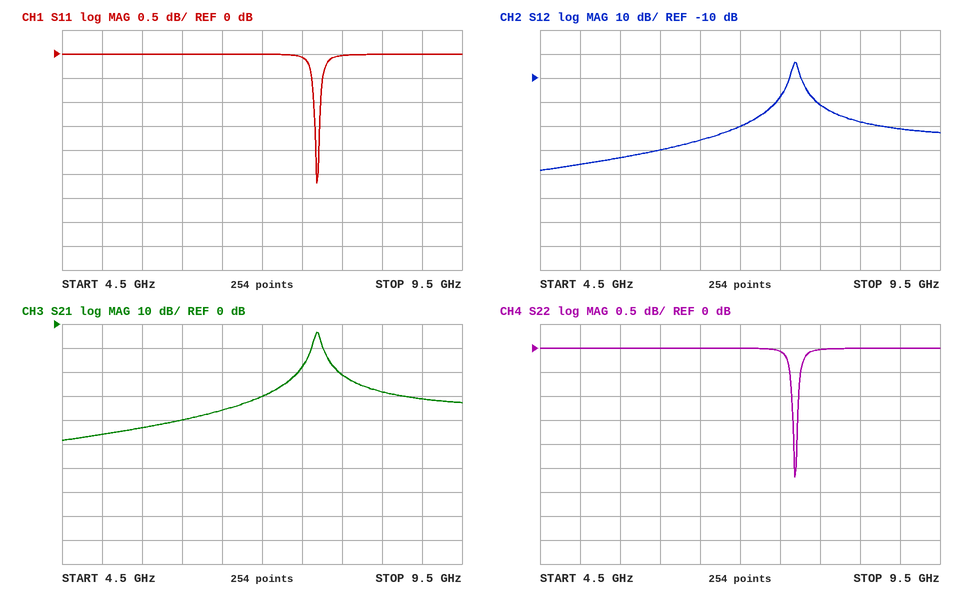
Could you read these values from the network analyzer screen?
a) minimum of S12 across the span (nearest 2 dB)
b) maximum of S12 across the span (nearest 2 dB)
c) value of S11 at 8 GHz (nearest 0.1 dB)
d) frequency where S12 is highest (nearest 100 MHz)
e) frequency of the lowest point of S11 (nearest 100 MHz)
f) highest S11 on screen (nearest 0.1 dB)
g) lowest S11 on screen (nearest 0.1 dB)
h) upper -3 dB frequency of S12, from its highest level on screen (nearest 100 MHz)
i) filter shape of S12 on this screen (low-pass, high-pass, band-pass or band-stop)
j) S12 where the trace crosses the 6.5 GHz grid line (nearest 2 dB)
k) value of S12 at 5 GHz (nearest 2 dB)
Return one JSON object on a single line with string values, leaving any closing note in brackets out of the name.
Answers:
{"minimum of S12 across the span": "-48 dB", "maximum of S12 across the span": "-4 dB", "value of S11 at 8 GHz": "0.0 dB", "frequency where S12 is highest": "7.7 GHz", "frequency of the lowest point of S11": "7.7 GHz", "highest S11 on screen": "0.0 dB", "lowest S11 on screen": "-2.7 dB", "upper -3 dB frequency of S12, from its highest level on screen": "7.7 GHz", "filter shape of S12 on this screen": "band-pass", "S12 where the trace crosses the 6.5 GHz grid line": "-36 dB", "value of S12 at 5 GHz": "-46 dB"}
